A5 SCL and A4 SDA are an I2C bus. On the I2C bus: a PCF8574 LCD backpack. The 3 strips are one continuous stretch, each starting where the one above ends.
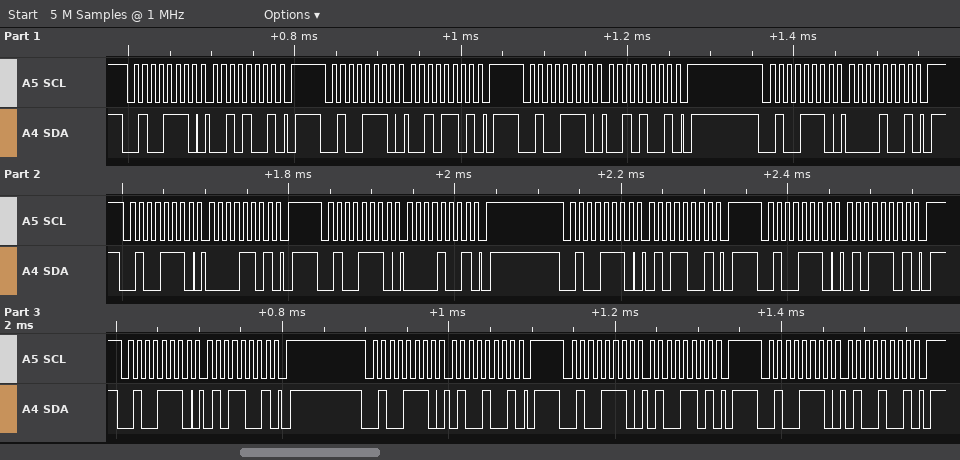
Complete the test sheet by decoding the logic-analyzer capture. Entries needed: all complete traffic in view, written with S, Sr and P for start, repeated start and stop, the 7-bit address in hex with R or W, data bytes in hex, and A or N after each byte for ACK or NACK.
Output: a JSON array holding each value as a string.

["S 27W A 29 A P S 27W A 2D A P S 27W A 29 A P S 27W A 09 A P S 27W A 0D A P S 27W A 09 A P S 27W A 59 A P S 27W A 5D A P S 27W A 59 A P S 27W A 49 A P S 27W A 4D A P S 27W A 49 A P"]
